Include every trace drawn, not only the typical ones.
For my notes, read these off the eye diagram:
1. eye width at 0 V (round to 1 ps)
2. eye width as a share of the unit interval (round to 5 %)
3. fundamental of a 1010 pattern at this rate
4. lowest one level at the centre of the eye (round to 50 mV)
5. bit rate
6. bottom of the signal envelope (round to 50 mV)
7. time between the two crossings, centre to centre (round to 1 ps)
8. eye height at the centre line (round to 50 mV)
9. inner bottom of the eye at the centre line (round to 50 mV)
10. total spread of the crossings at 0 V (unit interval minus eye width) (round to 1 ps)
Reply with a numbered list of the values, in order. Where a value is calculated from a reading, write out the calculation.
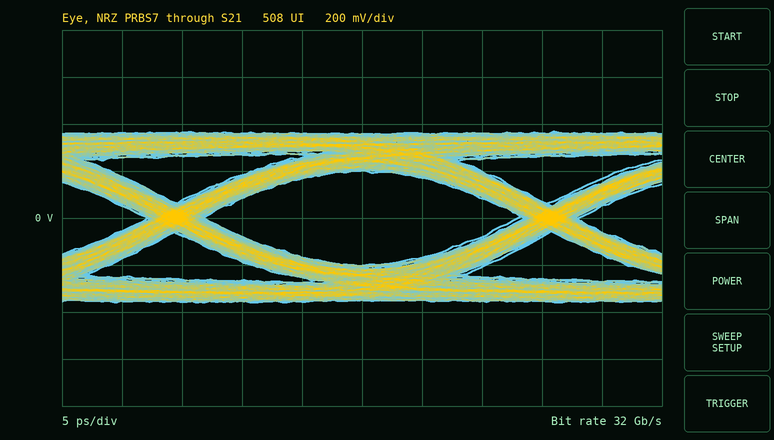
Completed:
1. 26 ps
2. 26 ps / 31 ps ≈ 83.9 %, so 85 % to the nearest 5 %
3. 16 GHz
4. 200 mV
5. 32 Gb/s
6. -350 mV
7. 31 ps
8. 400 mV
9. -200 mV
10. 5 ps
